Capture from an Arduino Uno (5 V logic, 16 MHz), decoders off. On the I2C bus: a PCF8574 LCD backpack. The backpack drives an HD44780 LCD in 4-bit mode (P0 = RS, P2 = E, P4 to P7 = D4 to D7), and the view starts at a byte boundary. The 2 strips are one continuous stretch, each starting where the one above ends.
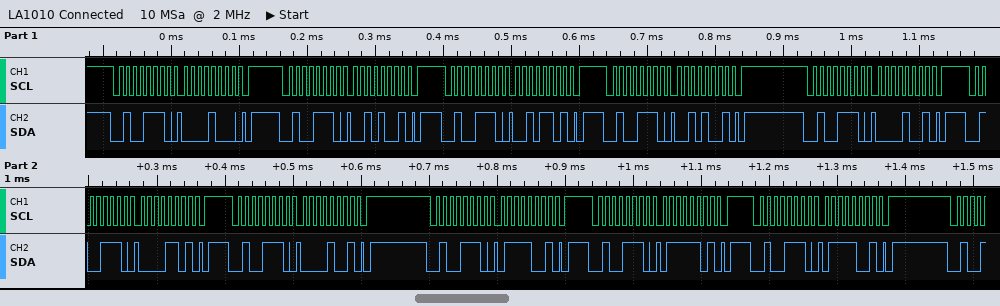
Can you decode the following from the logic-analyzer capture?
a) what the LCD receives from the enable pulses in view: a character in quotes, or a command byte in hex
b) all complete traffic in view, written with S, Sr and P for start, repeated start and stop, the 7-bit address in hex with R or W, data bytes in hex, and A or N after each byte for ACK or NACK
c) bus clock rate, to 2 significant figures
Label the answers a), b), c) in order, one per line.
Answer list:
a) ' '
b) S 27W A 08 A P S 27W A 29 A P S 27W A 2D A P S 27W A 29 A P S 27W A 09 A P S 27W A 0D A P S 27W A 09 A P S 27W A 79 A P S 27W A 7D A P S 27W A 79 A P
c) 100 kHz
